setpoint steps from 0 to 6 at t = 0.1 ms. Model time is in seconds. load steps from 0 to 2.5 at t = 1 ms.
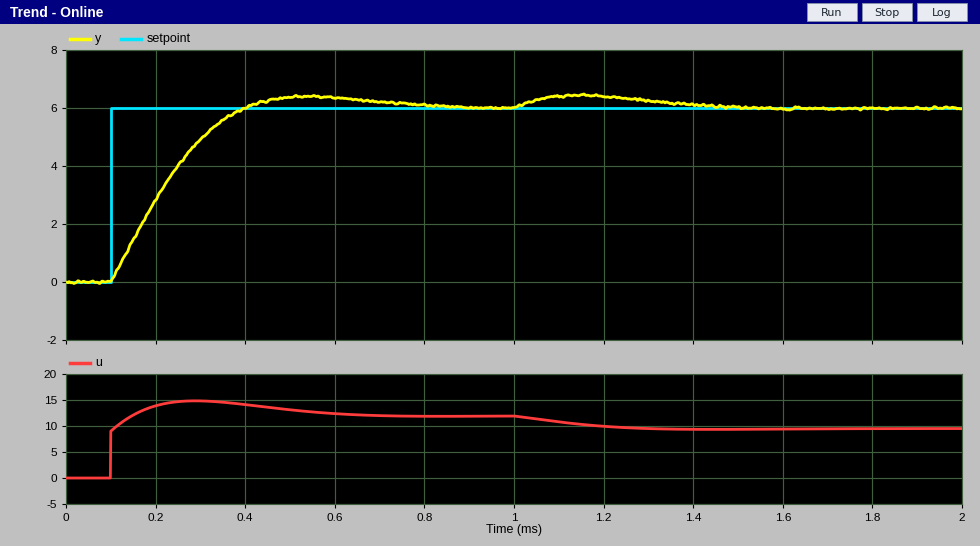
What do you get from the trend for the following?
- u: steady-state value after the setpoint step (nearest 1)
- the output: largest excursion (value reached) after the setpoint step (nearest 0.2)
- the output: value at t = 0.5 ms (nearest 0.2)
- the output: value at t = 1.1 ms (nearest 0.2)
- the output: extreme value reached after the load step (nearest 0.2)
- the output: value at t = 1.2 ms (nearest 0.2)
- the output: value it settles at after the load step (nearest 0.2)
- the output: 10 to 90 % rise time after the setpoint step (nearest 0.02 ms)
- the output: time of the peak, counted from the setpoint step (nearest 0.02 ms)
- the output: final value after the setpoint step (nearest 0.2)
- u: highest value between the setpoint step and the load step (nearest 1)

12
6.4
6.4
6.4
6.4
6.4
6.0
0.22 ms
0.44 ms
6.0
15
